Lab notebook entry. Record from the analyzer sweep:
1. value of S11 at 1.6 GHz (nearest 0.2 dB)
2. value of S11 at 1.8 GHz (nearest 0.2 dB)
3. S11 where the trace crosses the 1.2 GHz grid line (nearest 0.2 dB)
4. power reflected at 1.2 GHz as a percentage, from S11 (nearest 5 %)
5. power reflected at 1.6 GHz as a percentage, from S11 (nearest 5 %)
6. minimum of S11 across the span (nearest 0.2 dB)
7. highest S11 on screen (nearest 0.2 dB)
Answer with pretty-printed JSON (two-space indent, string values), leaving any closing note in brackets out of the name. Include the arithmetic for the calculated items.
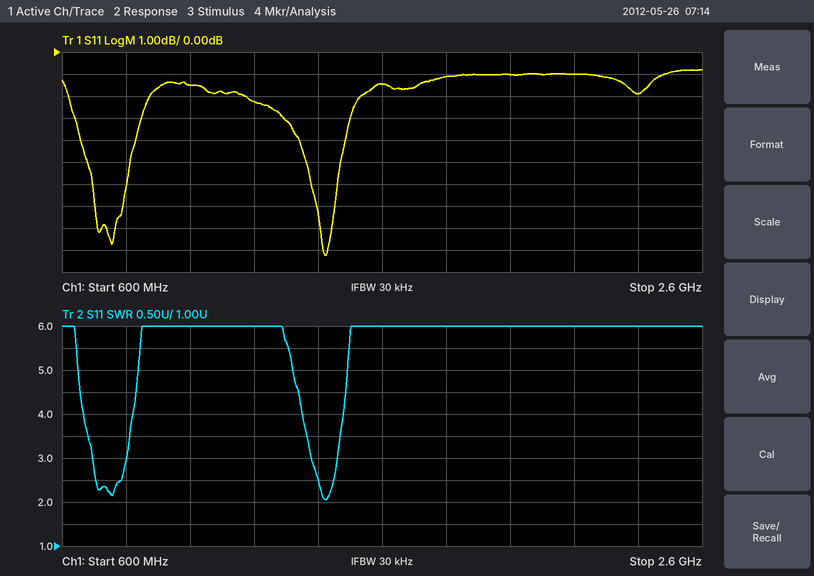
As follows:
{
  "value of S11 at 1.6 GHz": "-1.4 dB",
  "value of S11 at 1.8 GHz": "-1.2 dB",
  "S11 where the trace crosses the 1.2 GHz grid line": "-2.2 dB",
  "power reflected at 1.2 GHz as a percentage, from S11": "10^(-2.2/10) ≈ 60 %",
  "power reflected at 1.6 GHz as a percentage, from S11": "10^(-1.4/10) ≈ 72.4 %, so 70 % to the nearest 5 %",
  "minimum of S11 across the span": "-9.2 dB",
  "highest S11 on screen": "-0.8 dB"
}
